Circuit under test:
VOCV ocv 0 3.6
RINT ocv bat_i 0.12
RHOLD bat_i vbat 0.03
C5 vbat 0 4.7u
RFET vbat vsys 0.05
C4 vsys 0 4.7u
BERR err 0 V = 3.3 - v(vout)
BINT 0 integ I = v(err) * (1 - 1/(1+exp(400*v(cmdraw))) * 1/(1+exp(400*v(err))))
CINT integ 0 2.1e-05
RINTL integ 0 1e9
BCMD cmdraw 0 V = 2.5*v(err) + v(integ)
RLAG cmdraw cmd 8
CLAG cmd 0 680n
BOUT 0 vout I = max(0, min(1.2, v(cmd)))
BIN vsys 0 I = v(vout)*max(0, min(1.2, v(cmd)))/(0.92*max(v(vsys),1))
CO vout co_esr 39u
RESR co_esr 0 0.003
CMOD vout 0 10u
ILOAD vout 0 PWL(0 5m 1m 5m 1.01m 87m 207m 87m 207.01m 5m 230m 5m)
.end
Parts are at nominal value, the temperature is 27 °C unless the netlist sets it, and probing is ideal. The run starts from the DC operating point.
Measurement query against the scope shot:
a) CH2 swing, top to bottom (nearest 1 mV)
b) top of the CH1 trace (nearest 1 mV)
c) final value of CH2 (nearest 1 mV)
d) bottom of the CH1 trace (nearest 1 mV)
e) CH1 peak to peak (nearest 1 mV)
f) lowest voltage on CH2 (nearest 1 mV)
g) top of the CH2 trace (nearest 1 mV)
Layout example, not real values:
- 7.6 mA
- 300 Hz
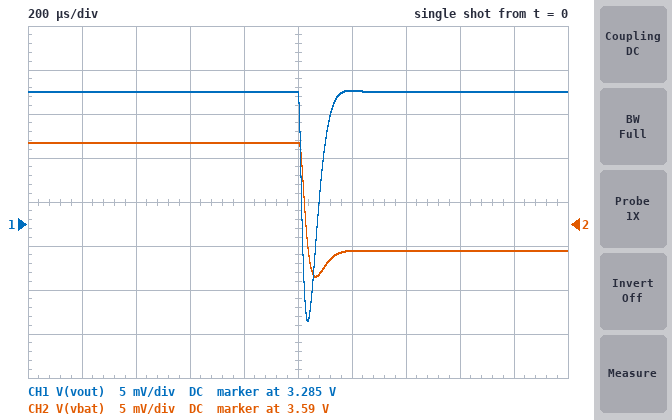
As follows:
- 15 mV
- 3.300 V
- 3.587 V
- 3.274 V
- 26 mV
- 3.584 V
- 3.599 V
